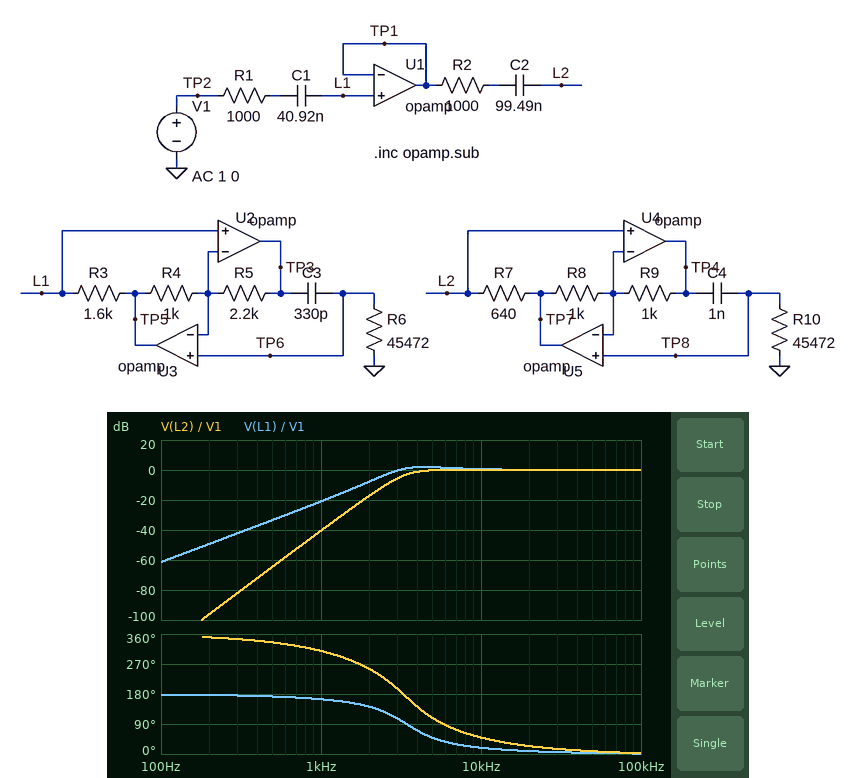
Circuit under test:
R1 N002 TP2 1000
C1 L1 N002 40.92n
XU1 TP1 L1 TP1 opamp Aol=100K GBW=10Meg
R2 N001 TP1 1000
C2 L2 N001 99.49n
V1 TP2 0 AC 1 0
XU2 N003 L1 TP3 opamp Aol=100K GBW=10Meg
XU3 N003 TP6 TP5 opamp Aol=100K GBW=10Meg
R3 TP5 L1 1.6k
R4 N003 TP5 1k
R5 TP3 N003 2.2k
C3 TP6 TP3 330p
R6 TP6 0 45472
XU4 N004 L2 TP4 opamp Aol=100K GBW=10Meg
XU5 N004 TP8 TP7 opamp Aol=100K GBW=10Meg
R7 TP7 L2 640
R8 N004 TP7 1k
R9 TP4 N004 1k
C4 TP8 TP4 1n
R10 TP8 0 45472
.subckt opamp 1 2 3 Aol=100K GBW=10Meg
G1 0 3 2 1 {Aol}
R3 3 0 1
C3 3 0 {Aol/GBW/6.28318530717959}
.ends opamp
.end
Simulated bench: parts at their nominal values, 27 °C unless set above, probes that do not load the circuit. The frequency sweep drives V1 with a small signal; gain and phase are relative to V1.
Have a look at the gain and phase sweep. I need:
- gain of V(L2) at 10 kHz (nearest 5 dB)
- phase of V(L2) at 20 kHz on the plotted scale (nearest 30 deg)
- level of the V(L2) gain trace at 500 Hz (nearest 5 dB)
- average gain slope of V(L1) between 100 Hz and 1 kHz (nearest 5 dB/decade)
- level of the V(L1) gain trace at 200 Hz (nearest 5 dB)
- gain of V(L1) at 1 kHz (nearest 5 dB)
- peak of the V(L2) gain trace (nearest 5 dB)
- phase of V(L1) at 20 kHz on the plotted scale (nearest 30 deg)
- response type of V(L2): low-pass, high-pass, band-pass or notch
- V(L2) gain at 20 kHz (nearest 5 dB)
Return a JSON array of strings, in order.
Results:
["0 dB", "30 deg", "-65 dB", "40 dB/decade", "-50 dB", "-20 dB", "0 dB", "0 deg", "high-pass", "0 dB"]
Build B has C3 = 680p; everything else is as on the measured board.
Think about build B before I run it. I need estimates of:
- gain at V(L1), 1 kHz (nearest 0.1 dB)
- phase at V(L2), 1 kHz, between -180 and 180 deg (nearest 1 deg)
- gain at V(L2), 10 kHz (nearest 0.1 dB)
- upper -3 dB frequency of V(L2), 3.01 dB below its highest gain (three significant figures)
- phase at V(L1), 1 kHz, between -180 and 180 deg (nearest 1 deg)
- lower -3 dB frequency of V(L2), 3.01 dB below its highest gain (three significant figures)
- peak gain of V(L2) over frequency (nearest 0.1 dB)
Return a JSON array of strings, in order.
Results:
["-13.8 dB", "-53 deg", "-0.1 dB", "2.13 MHz", "163 deg", "2.41 kHz", "0 dB"]
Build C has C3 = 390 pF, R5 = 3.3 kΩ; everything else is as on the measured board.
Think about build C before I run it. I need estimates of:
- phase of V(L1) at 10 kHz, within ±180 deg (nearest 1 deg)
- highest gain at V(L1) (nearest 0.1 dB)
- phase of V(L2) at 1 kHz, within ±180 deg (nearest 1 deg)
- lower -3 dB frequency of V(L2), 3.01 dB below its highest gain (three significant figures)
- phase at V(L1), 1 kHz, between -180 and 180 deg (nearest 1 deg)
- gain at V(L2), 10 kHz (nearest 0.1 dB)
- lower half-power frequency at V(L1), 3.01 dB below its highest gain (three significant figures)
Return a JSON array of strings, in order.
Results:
["10 deg", "4.1 dB", "-52 deg", "2.58 kHz", "163 deg", "-0.1 dB", "2.17 kHz"]
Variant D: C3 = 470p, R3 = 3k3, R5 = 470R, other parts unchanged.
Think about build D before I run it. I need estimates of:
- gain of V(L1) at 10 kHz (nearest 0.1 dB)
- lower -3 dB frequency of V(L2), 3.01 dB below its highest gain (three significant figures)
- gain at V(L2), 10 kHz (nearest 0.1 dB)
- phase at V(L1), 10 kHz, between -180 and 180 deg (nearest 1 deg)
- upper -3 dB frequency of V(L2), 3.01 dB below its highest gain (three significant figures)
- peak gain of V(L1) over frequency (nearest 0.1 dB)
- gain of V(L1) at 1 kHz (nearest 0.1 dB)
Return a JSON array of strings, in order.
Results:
["0.5 dB", "4.55 kHz", "0 dB", "30 deg", "1.95 MHz", "0.7 dB", "-25.2 dB"]
